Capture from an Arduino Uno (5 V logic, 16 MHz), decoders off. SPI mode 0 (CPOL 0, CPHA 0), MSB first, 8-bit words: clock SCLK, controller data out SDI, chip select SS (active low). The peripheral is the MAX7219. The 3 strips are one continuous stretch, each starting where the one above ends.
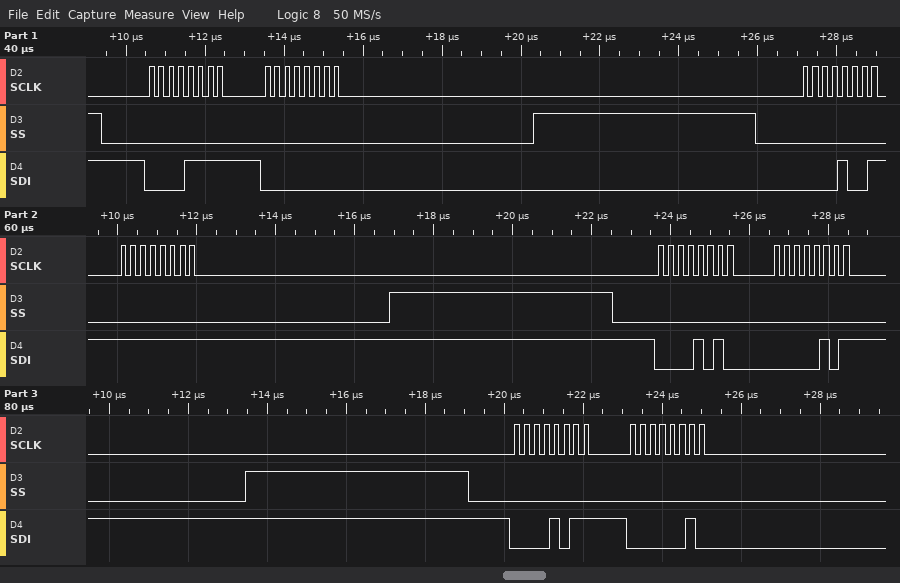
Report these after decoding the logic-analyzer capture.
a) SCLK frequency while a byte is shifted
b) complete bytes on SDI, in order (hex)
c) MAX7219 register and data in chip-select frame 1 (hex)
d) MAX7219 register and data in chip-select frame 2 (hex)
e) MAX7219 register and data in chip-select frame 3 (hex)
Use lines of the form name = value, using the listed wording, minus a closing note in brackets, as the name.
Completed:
SCLK frequency while a byte is shifted = 4 MHz
complete bytes on SDI, in order = 0x0F 0x00 0x09 0xFF 0x0A 0x05 0x0B 0x02
MAX7219 register and data in chip-select frame 1 = register 0xF, data 0x00
MAX7219 register and data in chip-select frame 2 = register 0x9, data 0xFF
MAX7219 register and data in chip-select frame 3 = register 0xA, data 0x05
